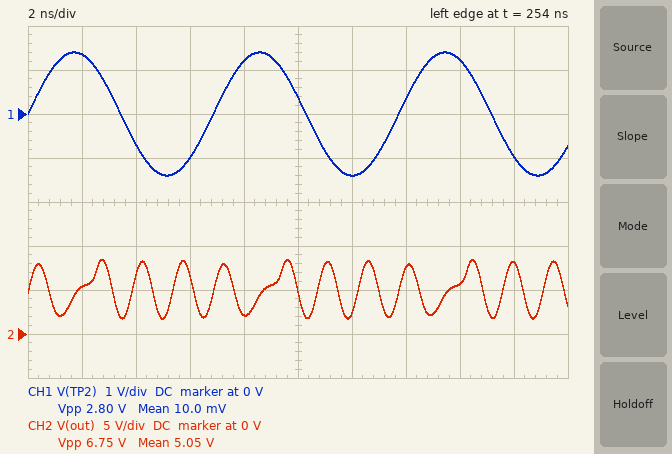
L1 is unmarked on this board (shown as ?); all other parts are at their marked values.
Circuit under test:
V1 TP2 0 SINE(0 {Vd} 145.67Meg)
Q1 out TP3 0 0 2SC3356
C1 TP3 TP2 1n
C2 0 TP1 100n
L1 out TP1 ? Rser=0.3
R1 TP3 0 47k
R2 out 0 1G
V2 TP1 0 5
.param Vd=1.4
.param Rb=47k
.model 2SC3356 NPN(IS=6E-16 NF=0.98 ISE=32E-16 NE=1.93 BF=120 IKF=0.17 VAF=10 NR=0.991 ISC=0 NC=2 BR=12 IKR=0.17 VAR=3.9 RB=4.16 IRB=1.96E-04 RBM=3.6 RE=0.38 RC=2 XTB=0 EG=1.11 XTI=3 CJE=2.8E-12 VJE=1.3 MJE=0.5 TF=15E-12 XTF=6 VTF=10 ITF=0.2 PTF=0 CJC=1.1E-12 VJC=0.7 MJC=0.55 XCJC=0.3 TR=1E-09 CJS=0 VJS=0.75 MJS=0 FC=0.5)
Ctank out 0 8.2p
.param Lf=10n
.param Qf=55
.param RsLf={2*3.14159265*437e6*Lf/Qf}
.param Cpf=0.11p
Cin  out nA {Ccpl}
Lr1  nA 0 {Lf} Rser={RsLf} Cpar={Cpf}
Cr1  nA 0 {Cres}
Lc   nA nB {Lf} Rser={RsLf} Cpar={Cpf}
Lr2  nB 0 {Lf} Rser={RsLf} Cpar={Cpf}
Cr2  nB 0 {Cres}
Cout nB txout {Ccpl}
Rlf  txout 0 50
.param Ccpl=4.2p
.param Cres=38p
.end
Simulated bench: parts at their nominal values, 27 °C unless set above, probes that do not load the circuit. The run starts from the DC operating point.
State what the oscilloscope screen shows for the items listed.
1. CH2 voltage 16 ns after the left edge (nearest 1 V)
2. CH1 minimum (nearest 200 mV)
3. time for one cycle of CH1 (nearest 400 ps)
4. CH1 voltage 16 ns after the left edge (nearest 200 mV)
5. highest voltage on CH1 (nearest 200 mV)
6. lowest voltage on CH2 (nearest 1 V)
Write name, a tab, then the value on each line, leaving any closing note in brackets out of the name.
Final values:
CH2 voltage 16 ns after the left edge	6 V
CH1 minimum	-1.4 V
time for one cycle of CH1	6.8 ns
CH1 voltage 16 ns after the left edge	1.2 V
highest voltage on CH1	1.4 V
lowest voltage on CH2	2 V
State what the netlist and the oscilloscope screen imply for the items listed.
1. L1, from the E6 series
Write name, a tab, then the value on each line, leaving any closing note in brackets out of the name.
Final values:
L1, from the E6 series	4.7 nH
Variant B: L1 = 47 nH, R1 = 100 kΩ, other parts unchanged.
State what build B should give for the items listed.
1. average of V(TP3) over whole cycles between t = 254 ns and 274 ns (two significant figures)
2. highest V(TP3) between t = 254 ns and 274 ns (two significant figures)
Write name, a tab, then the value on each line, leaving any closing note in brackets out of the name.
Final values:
average of V(TP3) over whole cycles between t = 254 ns and 274 ns	-440 mV
highest V(TP3) between t = 254 ns and 274 ns	950 mV
